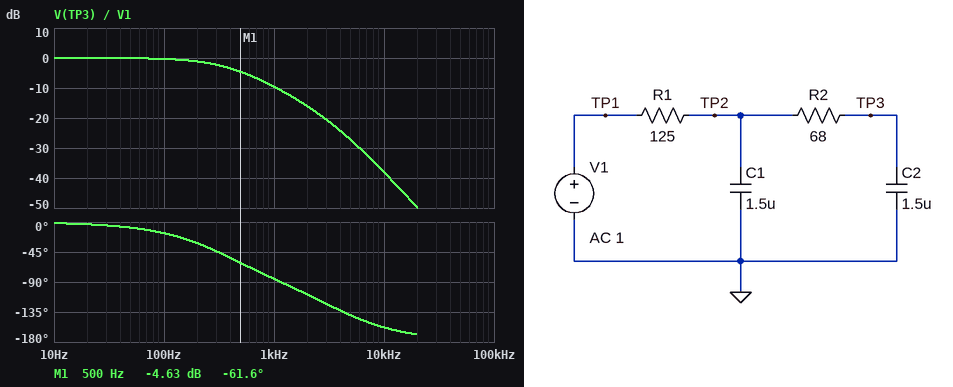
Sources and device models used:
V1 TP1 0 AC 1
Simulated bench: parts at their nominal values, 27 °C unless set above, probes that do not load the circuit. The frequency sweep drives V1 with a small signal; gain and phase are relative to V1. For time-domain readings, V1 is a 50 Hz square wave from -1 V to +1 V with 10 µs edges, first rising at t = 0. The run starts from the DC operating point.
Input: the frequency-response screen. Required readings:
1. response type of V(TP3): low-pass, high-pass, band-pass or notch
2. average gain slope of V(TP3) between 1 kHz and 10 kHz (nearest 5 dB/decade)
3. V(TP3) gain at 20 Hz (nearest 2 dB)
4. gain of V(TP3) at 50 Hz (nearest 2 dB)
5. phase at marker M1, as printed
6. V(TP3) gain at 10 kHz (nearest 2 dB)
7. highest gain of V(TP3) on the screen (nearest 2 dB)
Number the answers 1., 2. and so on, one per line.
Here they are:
1. low-pass
2. -30 dB/decade
3. 0 dB
4. 0 dB
5. -61.6 deg
6. -38 dB
7. 0 dB
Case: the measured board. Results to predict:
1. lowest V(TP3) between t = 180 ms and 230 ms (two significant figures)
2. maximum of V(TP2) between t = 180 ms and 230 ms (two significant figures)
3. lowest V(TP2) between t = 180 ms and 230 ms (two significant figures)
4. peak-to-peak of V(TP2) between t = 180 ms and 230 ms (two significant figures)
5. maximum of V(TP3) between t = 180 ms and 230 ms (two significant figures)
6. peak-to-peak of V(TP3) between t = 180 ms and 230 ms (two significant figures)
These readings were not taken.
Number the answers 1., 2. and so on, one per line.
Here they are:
1. -1.0 V
2. 1.0 V
3. -1.0 V
4. 2.0 V
5. 1.0 V
6. 2.0 V
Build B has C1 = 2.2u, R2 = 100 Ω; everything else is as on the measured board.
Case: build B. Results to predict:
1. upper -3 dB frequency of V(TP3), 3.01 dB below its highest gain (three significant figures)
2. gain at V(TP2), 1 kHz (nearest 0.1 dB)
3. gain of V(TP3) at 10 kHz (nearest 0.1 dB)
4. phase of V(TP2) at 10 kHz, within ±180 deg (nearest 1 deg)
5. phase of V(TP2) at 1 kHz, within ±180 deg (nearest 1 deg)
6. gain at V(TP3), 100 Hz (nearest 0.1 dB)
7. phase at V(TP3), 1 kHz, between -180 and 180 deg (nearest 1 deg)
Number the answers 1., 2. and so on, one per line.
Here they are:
1. 291 Hz
2. -9.1 dB
3. -44.4 dB
4. -83 deg
5. -56 deg
6. -0.5 dB
7. -99 deg
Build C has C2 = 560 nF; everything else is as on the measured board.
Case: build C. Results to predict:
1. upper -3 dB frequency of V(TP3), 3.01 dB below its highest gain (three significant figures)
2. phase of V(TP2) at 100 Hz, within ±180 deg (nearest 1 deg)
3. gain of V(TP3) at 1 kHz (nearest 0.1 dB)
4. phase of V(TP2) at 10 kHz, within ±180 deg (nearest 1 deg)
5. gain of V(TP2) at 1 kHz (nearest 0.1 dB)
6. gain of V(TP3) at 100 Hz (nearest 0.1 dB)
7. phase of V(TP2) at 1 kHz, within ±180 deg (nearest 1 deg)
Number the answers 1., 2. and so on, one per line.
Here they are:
1. 586 Hz
2. -9 deg
3. -6.0 dB
4. -78 deg
5. -5.7 dB
6. -0.1 dB
7. -55 deg
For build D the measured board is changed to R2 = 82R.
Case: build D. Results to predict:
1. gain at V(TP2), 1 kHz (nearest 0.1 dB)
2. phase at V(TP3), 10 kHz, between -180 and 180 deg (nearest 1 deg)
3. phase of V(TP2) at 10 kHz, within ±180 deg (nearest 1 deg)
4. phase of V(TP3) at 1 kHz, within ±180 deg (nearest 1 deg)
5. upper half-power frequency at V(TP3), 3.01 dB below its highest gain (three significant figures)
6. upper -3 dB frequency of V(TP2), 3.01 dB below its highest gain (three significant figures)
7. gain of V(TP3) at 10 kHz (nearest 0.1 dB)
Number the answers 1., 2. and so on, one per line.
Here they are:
1. -7.9 dB
2. -161 deg
3. -78 deg
4. -88 deg
5. 352 Hz
6. 381 Hz
7. -39.6 dB
